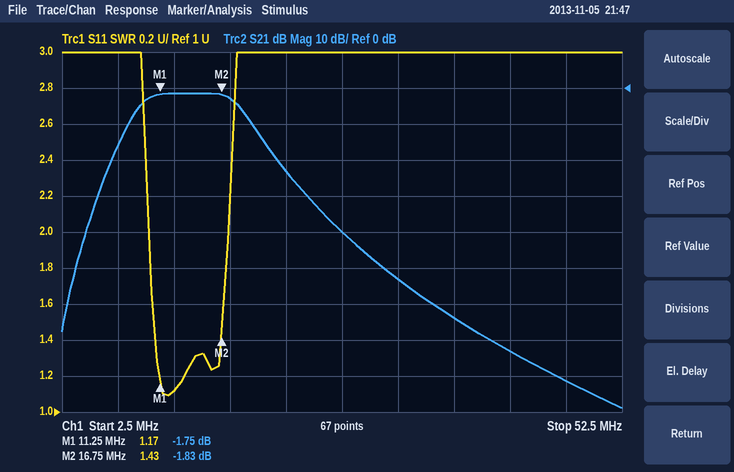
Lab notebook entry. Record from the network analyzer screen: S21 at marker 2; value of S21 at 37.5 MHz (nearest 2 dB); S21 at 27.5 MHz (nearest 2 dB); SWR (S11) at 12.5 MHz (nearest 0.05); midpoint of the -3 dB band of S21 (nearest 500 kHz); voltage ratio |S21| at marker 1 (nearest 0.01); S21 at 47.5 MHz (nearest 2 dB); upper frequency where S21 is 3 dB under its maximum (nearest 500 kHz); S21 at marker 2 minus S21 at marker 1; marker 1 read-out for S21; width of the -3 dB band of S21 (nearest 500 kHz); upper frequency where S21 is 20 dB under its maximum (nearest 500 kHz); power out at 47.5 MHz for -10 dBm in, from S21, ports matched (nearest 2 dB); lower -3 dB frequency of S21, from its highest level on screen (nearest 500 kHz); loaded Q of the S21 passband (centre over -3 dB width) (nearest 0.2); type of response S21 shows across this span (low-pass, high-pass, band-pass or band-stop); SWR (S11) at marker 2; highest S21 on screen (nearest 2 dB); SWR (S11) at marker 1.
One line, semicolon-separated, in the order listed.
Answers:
-1.83 dB; -64 dB; -40 dB; 1.10; 14.0 MHz; 0.82; -82 dB; 18.0 MHz; -0.08 dB; -1.75 dB; 8.5 MHz; 22.0 MHz; -92 dBm; 9.5 MHz; 1.6; band-pass; 1.43; -2 dB; 1.17
